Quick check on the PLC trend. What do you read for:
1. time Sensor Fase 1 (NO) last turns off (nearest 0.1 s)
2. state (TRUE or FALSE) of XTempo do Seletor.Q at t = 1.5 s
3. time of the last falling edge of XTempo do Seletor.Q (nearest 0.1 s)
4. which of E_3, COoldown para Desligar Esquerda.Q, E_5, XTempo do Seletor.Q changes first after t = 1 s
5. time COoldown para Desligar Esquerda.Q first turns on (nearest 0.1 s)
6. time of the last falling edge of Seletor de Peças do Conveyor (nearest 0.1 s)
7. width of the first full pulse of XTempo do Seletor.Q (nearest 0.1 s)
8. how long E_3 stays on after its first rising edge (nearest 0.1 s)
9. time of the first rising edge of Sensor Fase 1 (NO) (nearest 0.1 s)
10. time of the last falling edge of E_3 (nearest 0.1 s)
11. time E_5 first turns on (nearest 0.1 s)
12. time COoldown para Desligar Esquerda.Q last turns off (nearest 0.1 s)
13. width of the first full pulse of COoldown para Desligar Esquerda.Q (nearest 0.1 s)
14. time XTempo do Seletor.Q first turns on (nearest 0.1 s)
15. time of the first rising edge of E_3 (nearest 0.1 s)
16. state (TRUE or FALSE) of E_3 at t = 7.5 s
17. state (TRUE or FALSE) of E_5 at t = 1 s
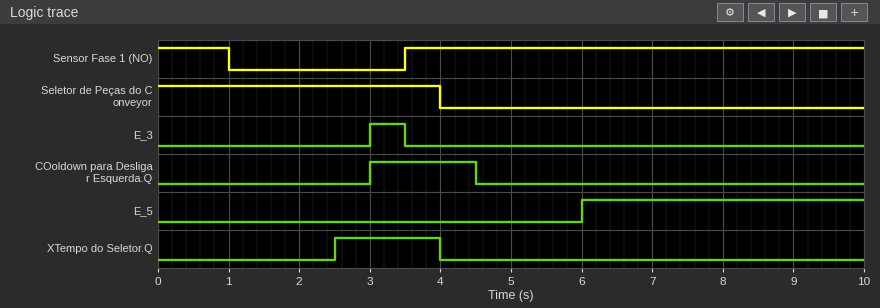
1.0 s
FALSE
4.0 s
XTempo do Seletor.Q
3.0 s
4.0 s
1.5 s
0.5 s
3.5 s
3.5 s
6.0 s
4.5 s
1.5 s
2.5 s
3.0 s
FALSE
FALSE
